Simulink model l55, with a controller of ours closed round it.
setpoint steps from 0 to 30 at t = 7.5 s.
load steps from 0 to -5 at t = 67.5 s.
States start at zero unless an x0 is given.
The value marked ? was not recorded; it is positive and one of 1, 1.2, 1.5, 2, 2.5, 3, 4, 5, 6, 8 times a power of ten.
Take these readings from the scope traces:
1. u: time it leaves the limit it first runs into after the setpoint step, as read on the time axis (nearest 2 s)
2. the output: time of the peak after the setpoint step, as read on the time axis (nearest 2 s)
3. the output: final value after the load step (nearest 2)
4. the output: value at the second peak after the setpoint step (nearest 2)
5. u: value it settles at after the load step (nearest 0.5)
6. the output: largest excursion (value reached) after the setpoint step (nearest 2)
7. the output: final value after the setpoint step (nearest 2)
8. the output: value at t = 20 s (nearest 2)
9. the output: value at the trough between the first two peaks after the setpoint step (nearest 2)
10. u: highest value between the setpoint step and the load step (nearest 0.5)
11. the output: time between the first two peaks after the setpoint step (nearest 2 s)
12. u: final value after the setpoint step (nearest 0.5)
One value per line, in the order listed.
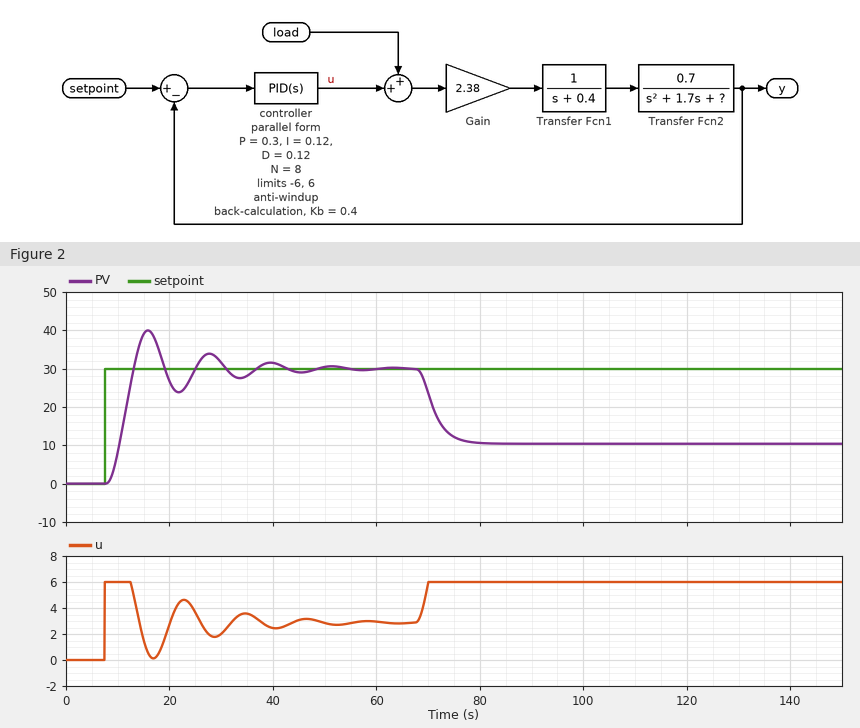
12 s
16 s
10
34
6.0
40
30
26
24
6.0
12 s
3.0
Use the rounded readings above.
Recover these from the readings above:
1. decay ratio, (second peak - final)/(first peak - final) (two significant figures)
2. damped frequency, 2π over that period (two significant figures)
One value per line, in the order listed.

0.40
0.52 rad/s
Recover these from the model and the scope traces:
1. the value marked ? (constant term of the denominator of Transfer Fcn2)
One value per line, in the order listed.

0.4
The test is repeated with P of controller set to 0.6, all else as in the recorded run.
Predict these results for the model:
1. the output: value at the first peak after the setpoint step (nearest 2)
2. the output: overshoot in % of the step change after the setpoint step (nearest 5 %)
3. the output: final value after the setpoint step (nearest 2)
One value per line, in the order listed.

32
10 %
30
